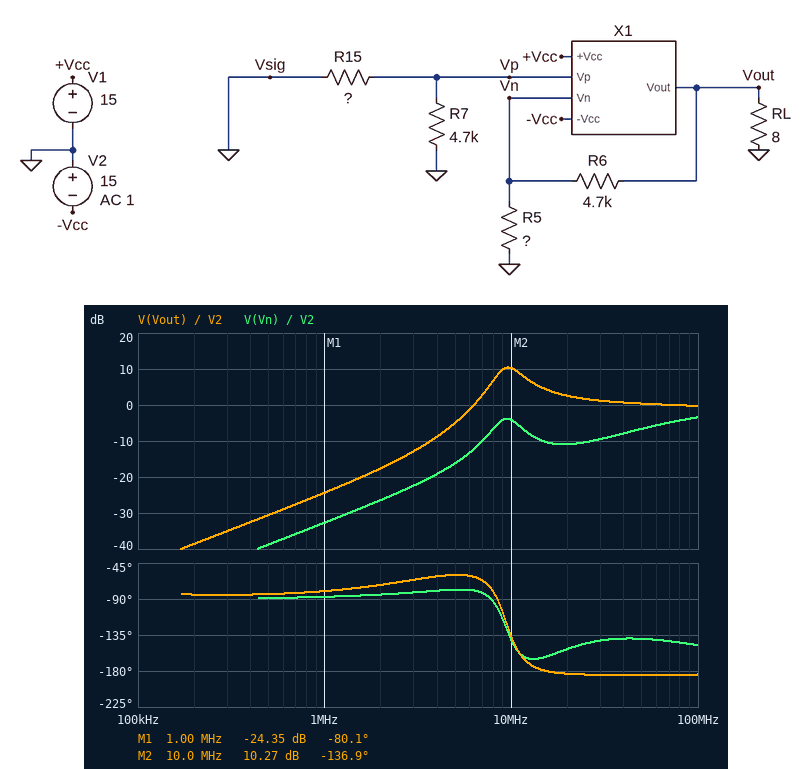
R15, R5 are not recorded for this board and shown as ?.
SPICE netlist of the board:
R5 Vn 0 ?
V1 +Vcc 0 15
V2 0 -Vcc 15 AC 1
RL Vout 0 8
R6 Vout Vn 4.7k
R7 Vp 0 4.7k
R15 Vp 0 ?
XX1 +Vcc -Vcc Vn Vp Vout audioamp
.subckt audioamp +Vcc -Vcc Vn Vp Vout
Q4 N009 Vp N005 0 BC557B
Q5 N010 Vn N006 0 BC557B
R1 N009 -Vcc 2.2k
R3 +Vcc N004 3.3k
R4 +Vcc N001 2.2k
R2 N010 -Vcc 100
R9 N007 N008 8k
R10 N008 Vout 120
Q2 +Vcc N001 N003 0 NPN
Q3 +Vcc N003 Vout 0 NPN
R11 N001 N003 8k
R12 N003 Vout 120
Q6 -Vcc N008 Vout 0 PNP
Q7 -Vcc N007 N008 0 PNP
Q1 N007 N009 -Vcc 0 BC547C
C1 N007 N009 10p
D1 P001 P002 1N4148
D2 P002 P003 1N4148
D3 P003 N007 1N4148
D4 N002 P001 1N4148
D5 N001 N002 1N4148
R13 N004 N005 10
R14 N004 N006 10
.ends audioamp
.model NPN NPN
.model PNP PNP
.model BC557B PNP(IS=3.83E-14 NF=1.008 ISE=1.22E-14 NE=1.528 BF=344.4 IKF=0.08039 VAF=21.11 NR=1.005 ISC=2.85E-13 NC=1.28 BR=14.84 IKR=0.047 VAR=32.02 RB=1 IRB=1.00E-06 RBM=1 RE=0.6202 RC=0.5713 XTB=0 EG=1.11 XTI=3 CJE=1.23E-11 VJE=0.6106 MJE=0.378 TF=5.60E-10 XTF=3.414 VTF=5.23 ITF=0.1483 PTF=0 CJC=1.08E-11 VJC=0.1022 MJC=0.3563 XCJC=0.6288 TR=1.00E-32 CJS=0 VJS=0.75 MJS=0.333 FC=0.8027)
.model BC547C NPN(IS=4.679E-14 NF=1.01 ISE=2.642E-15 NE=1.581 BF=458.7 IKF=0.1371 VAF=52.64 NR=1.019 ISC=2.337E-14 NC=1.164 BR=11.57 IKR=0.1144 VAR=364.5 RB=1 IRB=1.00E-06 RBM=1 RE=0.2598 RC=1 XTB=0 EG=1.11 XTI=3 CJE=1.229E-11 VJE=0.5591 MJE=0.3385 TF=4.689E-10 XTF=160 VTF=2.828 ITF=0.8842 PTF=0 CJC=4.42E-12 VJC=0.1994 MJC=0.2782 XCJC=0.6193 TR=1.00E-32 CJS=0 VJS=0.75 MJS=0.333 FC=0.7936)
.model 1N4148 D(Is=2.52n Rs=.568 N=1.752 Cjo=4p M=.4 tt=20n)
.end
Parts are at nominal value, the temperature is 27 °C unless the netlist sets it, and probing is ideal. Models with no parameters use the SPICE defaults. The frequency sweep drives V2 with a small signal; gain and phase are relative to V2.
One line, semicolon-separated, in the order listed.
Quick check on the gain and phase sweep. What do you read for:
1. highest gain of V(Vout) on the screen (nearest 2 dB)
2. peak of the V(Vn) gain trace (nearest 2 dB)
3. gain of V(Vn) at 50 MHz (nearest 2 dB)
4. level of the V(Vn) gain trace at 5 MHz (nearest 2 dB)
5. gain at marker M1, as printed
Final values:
10 dB; -4 dB; -6 dB; -16 dB; -24.35 dB
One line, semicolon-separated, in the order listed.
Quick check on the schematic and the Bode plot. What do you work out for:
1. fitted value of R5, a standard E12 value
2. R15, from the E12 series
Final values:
1.2 kΩ; 1.5 kΩ
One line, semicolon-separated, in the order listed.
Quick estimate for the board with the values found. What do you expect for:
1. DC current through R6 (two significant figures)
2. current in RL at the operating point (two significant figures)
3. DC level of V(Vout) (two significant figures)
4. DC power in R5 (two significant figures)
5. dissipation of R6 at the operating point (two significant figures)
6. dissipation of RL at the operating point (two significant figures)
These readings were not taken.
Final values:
96 µA; 70 mA; -560 mV; 9.4 µW; 43 µW; 39 mW
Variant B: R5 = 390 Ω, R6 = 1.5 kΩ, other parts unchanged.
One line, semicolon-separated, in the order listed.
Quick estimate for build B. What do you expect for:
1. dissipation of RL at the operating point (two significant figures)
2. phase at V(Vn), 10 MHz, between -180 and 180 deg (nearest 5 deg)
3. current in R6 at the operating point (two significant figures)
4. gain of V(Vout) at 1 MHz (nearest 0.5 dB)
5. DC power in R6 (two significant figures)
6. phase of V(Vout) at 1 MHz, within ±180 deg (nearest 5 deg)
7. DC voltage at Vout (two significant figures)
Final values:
35 mW; -130 deg; 280 µA; -20.5 dB; 120 µW; -85 deg; -530 mV
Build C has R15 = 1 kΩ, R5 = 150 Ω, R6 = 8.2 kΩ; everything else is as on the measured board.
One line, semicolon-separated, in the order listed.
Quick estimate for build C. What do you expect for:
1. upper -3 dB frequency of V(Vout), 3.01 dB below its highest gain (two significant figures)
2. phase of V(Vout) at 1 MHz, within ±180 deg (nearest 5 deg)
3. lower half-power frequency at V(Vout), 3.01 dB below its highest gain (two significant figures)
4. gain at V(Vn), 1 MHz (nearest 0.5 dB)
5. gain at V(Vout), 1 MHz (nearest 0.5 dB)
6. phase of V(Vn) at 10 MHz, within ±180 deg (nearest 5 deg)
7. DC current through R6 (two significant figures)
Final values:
11 MHz; -110 deg; 1.8 MHz; -35.0 dB; -0.5 dB; -155 deg; 710 µA
